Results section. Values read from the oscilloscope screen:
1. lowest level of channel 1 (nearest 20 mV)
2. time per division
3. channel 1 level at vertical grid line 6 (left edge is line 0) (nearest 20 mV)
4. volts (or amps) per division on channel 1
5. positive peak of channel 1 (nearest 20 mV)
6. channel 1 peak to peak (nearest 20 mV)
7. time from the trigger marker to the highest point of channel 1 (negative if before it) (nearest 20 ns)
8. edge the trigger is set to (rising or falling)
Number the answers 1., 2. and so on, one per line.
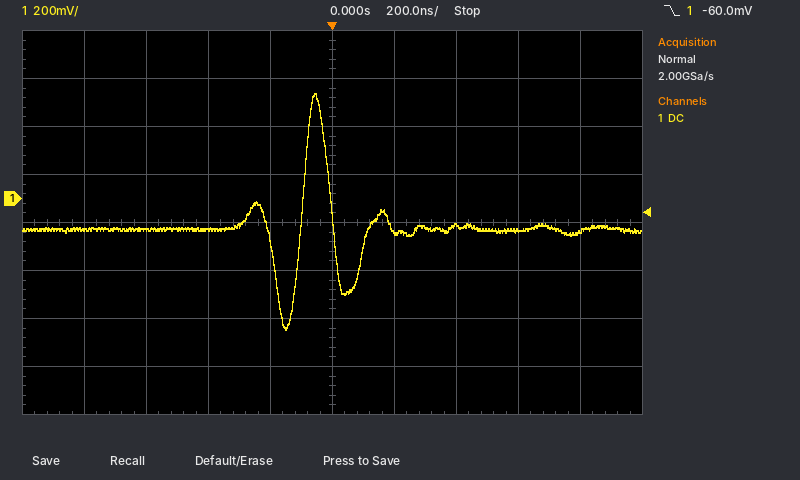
1. -540 mV
2. 200 ns
3. -140 mV
4. 200 mV
5. 440 mV
6. 980 mV
7. -60 ns
8. falling
